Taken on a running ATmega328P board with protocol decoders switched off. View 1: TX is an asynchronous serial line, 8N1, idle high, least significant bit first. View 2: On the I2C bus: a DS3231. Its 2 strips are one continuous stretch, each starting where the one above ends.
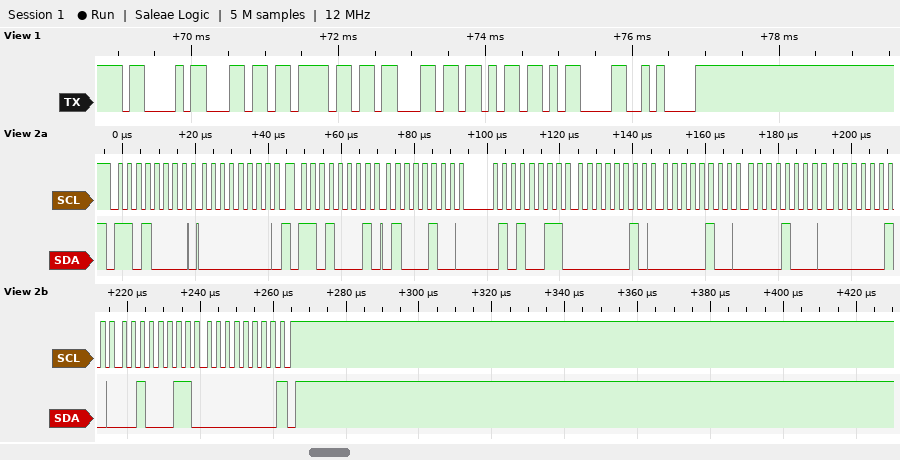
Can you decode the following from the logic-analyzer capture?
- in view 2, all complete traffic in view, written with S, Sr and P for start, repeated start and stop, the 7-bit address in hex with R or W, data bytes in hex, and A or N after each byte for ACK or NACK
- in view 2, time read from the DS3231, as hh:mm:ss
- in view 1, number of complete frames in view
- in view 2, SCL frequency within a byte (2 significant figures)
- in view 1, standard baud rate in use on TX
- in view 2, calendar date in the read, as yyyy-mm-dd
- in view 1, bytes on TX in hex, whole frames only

S 68W A 00 A Sr 68R A 44 A 53 A 02 A 04 A 08 A 02 A 23 A 00 N P
02:53:44
7
400 kHz
9600 baud
2023-02-08
43 6C 6F 63 6B 0D 0A
